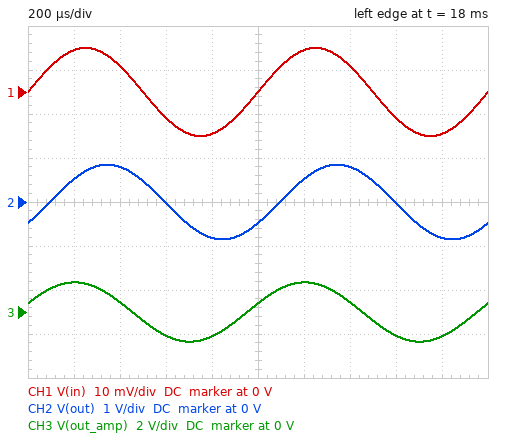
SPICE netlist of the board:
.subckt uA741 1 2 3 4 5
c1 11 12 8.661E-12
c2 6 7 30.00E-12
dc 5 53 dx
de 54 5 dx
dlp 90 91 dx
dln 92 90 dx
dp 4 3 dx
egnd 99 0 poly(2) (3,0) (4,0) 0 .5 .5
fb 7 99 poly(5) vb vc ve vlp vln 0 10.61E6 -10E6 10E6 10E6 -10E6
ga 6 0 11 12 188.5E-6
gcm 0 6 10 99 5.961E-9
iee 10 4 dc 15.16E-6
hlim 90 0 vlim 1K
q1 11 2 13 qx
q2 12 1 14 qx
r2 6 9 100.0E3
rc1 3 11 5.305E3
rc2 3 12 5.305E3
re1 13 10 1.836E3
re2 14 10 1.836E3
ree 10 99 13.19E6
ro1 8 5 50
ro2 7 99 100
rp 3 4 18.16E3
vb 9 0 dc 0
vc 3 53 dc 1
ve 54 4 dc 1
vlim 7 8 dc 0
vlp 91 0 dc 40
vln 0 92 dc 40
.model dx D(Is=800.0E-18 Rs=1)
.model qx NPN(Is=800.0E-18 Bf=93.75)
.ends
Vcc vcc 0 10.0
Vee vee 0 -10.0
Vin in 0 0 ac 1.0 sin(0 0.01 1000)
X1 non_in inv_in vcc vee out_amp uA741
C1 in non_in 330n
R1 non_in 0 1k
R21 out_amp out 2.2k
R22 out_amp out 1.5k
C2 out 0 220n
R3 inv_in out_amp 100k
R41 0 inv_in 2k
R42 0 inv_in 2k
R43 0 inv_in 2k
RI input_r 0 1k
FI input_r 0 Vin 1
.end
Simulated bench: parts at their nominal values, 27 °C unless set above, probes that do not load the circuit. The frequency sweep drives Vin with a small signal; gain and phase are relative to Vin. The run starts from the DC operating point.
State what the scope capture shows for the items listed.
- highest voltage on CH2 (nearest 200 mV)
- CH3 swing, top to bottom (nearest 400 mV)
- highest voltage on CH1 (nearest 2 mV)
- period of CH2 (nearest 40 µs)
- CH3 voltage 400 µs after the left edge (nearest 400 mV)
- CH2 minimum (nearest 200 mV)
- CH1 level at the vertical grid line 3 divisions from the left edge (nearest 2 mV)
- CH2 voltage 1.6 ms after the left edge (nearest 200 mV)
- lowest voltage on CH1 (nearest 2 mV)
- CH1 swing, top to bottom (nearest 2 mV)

800 mV
2.8 V
10 mV
1.00 ms
400 mV
-800 mV
-6 mV
0 V
-10 mV
20 mV
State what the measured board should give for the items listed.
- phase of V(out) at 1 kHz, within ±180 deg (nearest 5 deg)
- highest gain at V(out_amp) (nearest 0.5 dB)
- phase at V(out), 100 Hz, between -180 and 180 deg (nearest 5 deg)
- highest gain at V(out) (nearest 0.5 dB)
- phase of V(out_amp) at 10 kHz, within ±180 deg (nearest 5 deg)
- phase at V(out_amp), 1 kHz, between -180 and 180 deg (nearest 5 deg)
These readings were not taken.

-35 deg
43.0 dB
70 deg
39.5 dB
-55 deg
15 deg
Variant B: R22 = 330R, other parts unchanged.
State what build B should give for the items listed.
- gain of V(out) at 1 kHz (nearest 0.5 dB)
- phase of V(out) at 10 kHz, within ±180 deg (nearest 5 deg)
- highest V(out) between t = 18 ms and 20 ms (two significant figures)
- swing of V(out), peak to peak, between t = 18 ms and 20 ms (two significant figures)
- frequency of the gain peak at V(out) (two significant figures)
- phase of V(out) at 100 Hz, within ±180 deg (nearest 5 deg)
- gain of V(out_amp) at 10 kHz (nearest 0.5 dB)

42.0 dB
-135 deg
1.3 V
2.5 V
1.1 kHz
75 deg
37.5 dB
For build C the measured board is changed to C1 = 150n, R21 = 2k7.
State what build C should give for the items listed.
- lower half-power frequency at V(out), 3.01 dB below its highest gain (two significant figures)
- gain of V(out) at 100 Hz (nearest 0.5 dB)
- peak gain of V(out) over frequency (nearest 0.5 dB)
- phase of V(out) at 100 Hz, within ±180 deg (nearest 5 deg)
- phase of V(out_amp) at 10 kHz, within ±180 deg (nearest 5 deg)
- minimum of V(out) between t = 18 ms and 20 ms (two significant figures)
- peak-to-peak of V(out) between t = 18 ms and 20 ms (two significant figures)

360 Hz
23.0 dB
36.0 dB
75 deg
-50 deg
-620 mV
1.2 V
